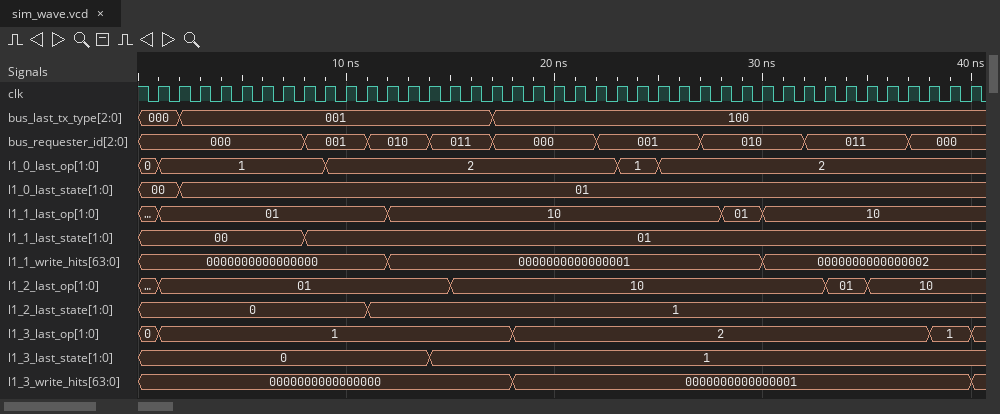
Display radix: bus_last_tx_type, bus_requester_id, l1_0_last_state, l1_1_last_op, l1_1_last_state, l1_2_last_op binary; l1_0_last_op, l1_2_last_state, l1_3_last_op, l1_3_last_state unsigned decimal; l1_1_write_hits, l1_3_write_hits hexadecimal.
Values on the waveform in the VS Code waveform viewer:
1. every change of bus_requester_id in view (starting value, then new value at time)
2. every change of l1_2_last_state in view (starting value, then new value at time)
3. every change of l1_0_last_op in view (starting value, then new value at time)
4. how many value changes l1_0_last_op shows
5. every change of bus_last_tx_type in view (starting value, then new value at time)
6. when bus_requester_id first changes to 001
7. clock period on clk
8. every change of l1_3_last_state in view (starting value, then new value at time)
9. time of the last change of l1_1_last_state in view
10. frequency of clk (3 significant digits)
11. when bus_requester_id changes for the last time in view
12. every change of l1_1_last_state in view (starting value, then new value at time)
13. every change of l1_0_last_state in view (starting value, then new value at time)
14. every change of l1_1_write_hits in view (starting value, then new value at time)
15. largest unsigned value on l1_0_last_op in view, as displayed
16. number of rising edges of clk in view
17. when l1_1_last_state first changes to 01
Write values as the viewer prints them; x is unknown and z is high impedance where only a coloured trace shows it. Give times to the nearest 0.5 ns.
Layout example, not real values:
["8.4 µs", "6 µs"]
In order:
["000, 001 at 8 ns, 010 at 11 ns, 011 at 14 ns, 000 at 17 ns, 001 at 22 ns, 010 at 27 ns, 011 at 32 ns, 000 at 37 ns", "0, 1 at 11 ns", "0, 1 at 1 ns, 2 at 9 ns, 1 at 23 ns, 2 at 25 ns", "4", "000, 001 at 2 ns, 100 at 17 ns", "8 ns", "1 ns", "0, 1 at 14 ns", "8 ns", "1.00 GHz", "37 ns", "00, 01 at 8 ns", "00, 01 at 2 ns", "0000000000000000, 0000000000000001 at 12 ns, 0000000000000002 at 30 ns", "2", "40", "8 ns"]
